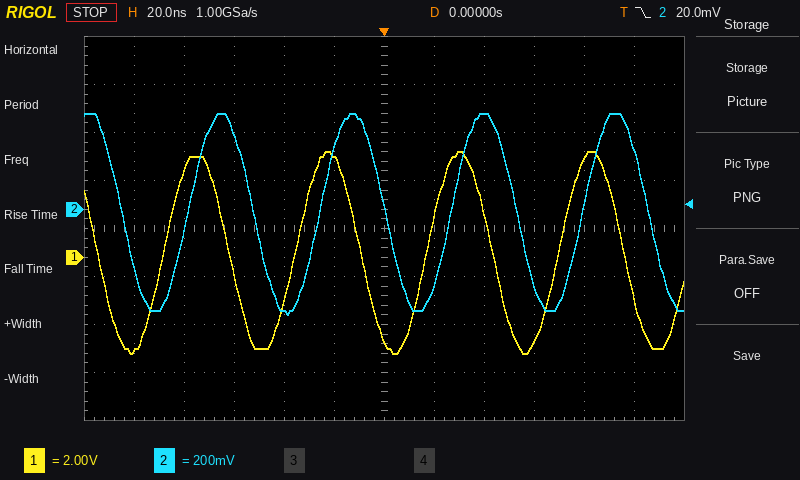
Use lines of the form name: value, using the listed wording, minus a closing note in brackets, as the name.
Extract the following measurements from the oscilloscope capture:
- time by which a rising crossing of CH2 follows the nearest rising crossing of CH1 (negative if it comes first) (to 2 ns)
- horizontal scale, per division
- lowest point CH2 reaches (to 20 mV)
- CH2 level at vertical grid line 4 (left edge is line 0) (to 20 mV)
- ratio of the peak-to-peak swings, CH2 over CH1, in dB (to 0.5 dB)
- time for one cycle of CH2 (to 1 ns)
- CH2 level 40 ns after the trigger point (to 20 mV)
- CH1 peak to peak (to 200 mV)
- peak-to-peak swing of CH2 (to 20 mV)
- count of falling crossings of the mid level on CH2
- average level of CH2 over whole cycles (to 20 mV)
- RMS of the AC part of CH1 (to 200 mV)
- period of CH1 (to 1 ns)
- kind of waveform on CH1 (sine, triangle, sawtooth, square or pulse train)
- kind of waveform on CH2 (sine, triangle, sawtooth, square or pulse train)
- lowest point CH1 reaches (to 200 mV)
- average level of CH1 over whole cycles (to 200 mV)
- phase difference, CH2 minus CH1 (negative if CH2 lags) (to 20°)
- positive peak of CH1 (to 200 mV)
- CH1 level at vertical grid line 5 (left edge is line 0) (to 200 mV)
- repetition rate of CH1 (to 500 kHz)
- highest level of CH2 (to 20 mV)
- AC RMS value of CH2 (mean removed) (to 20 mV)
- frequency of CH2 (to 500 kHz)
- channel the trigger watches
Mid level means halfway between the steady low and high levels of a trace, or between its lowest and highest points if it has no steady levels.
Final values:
time by which a rising crossing of CH2 follows the nearest rising crossing of CH1 (negative if it comes first): +10 ns
horizontal scale, per division: 20 ns
lowest point CH2 reaches: -440 mV
CH2 level at vertical grid line 4 (left edge is line 0): -420 mV
ratio of the peak-to-peak swings, CH2 over CH1, in dB: -20.0 dB
time for one cycle of CH2: 53 ns
CH2 level 40 ns after the trigger point: 400 mV
CH1 peak to peak: 8.4 V
peak-to-peak swing of CH2: 840 mV
count of falling crossings of the mid level on CH2: 5
average level of CH2 over whole cycles: -20 mV
RMS of the AC part of CH1: 3.0 V
period of CH1: 53 ns
kind of waveform on CH1: sine
kind of waveform on CH2: sine
lowest point CH1 reaches: -4.0 V
average level of CH1 over whole cycles: 200 mV
phase difference, CH2 minus CH1 (negative if CH2 lags): -60°
positive peak of CH1: 4.4 V
CH1 level at vertical grid line 5 (left edge is line 0): 4.2 V
repetition rate of CH1: 19.0 MHz
highest level of CH2: 400 mV
AC RMS value of CH2 (mean removed): 300 mV
frequency of CH2: 19.0 MHz
channel the trigger watches: CH2
